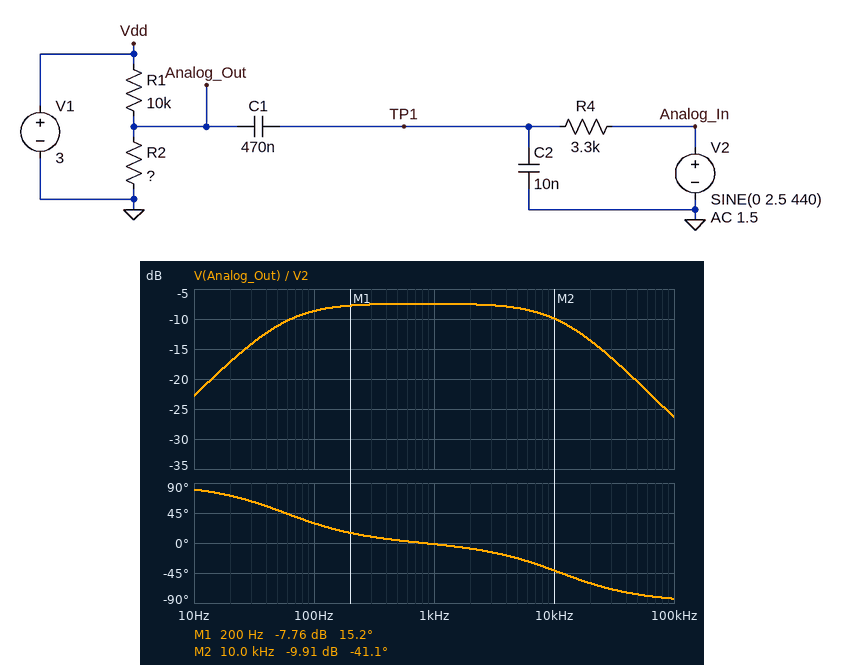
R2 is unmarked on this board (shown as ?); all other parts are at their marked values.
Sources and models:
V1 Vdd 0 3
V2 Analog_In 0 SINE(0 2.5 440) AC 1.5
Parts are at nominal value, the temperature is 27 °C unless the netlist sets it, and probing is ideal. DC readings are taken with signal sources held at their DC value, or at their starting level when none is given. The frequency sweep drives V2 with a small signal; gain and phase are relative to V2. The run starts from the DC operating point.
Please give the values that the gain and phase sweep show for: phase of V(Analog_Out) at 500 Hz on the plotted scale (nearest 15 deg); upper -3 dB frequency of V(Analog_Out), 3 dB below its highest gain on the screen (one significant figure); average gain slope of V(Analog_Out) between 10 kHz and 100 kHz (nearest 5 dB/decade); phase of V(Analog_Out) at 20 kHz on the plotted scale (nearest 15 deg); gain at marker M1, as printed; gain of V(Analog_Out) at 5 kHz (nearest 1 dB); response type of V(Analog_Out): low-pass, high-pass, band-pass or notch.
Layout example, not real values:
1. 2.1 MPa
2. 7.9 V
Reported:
1. 0 deg
2. 10 kHz
3. -15 dB/decade
4. -60 deg
5. -7.76 dB
6. -8 dB
7. band-pass
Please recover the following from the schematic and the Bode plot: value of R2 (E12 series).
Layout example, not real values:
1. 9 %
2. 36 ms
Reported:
1. 3.3 kΩ
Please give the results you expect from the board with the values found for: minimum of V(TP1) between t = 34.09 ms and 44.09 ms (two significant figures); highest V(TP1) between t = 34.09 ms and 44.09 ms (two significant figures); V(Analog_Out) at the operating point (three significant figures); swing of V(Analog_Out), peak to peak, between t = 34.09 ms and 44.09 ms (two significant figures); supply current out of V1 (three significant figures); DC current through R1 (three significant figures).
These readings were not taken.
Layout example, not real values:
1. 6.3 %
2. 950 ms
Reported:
1. -1.1 V
2. 1.1 V
3. 744 mV
4. 2.1 V
5. 226 µA
6. 226 µA
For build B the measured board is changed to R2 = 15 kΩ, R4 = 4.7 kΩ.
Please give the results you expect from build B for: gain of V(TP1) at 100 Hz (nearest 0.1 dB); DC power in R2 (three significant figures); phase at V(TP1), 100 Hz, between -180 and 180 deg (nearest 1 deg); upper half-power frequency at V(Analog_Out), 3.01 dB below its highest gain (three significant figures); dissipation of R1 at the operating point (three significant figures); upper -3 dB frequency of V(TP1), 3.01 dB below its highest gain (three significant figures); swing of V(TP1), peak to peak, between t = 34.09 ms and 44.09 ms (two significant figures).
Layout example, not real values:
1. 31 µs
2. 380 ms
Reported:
1. -4.3 dB
2. 216 µW
3. -13 deg
4. 6.13 kHz
5. 144 µW
6. 51.4 Hz
7. 2.8 V
